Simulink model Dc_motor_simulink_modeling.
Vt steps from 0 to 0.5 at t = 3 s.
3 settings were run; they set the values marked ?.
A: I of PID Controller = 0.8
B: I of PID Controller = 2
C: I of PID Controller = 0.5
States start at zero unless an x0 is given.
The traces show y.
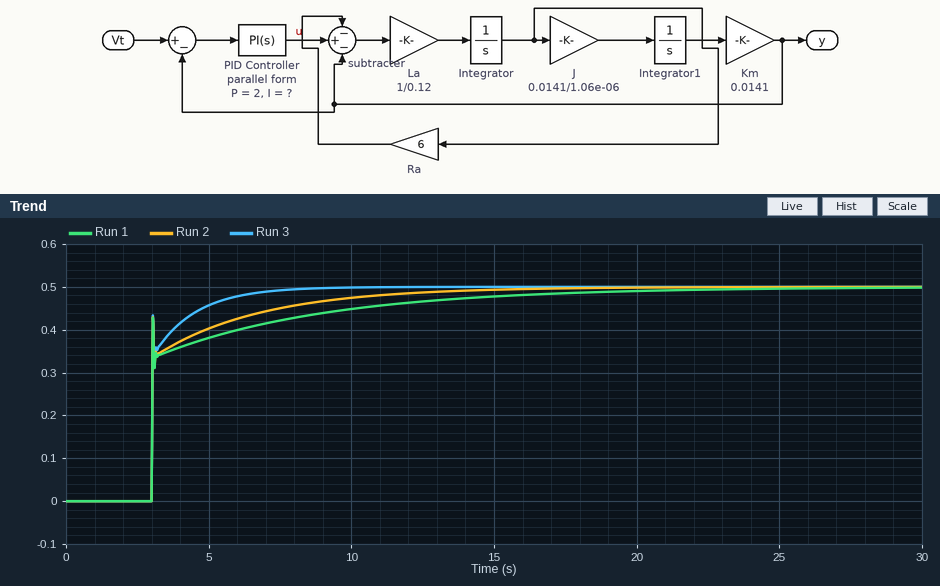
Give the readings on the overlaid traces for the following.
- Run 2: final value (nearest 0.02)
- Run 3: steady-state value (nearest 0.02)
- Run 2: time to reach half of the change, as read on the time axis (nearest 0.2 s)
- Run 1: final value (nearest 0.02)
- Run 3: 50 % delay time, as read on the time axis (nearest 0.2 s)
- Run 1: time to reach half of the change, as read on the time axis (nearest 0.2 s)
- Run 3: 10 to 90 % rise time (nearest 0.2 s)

0.50
0.50
3.0 s
0.50
3.0 s
3.0 s
1.8 s
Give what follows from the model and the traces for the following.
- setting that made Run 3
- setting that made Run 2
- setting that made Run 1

B
A
C
